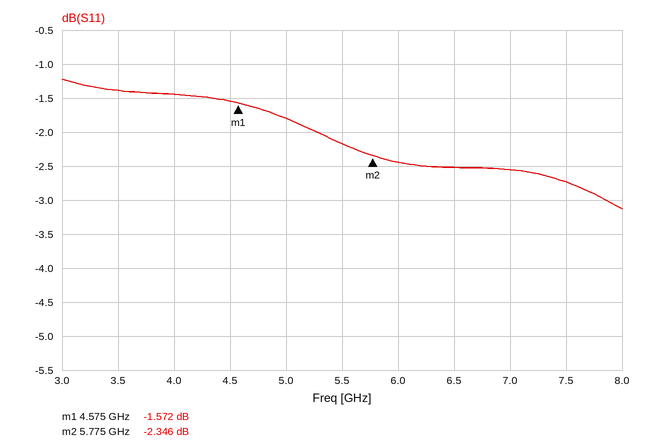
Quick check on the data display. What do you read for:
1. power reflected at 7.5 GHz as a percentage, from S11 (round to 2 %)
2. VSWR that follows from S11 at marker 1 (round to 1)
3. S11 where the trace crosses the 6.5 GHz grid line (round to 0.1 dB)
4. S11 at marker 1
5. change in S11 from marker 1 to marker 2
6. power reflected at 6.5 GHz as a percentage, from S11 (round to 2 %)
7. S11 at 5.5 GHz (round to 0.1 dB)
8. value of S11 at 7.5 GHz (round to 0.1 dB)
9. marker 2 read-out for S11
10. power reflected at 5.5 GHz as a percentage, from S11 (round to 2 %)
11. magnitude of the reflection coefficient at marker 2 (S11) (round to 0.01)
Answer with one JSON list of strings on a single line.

["54 %", "11", "-2.5 dB", "-1.572 dB", "-0.774 dB", "56 %", "-2.2 dB", "-2.7 dB", "-2.346 dB", "60 %", "0.76"]
